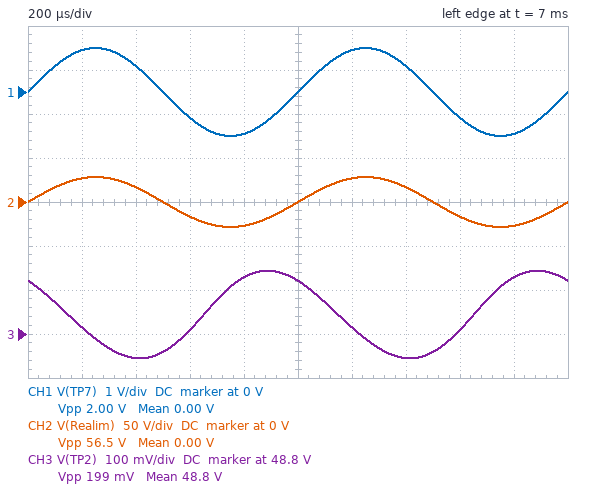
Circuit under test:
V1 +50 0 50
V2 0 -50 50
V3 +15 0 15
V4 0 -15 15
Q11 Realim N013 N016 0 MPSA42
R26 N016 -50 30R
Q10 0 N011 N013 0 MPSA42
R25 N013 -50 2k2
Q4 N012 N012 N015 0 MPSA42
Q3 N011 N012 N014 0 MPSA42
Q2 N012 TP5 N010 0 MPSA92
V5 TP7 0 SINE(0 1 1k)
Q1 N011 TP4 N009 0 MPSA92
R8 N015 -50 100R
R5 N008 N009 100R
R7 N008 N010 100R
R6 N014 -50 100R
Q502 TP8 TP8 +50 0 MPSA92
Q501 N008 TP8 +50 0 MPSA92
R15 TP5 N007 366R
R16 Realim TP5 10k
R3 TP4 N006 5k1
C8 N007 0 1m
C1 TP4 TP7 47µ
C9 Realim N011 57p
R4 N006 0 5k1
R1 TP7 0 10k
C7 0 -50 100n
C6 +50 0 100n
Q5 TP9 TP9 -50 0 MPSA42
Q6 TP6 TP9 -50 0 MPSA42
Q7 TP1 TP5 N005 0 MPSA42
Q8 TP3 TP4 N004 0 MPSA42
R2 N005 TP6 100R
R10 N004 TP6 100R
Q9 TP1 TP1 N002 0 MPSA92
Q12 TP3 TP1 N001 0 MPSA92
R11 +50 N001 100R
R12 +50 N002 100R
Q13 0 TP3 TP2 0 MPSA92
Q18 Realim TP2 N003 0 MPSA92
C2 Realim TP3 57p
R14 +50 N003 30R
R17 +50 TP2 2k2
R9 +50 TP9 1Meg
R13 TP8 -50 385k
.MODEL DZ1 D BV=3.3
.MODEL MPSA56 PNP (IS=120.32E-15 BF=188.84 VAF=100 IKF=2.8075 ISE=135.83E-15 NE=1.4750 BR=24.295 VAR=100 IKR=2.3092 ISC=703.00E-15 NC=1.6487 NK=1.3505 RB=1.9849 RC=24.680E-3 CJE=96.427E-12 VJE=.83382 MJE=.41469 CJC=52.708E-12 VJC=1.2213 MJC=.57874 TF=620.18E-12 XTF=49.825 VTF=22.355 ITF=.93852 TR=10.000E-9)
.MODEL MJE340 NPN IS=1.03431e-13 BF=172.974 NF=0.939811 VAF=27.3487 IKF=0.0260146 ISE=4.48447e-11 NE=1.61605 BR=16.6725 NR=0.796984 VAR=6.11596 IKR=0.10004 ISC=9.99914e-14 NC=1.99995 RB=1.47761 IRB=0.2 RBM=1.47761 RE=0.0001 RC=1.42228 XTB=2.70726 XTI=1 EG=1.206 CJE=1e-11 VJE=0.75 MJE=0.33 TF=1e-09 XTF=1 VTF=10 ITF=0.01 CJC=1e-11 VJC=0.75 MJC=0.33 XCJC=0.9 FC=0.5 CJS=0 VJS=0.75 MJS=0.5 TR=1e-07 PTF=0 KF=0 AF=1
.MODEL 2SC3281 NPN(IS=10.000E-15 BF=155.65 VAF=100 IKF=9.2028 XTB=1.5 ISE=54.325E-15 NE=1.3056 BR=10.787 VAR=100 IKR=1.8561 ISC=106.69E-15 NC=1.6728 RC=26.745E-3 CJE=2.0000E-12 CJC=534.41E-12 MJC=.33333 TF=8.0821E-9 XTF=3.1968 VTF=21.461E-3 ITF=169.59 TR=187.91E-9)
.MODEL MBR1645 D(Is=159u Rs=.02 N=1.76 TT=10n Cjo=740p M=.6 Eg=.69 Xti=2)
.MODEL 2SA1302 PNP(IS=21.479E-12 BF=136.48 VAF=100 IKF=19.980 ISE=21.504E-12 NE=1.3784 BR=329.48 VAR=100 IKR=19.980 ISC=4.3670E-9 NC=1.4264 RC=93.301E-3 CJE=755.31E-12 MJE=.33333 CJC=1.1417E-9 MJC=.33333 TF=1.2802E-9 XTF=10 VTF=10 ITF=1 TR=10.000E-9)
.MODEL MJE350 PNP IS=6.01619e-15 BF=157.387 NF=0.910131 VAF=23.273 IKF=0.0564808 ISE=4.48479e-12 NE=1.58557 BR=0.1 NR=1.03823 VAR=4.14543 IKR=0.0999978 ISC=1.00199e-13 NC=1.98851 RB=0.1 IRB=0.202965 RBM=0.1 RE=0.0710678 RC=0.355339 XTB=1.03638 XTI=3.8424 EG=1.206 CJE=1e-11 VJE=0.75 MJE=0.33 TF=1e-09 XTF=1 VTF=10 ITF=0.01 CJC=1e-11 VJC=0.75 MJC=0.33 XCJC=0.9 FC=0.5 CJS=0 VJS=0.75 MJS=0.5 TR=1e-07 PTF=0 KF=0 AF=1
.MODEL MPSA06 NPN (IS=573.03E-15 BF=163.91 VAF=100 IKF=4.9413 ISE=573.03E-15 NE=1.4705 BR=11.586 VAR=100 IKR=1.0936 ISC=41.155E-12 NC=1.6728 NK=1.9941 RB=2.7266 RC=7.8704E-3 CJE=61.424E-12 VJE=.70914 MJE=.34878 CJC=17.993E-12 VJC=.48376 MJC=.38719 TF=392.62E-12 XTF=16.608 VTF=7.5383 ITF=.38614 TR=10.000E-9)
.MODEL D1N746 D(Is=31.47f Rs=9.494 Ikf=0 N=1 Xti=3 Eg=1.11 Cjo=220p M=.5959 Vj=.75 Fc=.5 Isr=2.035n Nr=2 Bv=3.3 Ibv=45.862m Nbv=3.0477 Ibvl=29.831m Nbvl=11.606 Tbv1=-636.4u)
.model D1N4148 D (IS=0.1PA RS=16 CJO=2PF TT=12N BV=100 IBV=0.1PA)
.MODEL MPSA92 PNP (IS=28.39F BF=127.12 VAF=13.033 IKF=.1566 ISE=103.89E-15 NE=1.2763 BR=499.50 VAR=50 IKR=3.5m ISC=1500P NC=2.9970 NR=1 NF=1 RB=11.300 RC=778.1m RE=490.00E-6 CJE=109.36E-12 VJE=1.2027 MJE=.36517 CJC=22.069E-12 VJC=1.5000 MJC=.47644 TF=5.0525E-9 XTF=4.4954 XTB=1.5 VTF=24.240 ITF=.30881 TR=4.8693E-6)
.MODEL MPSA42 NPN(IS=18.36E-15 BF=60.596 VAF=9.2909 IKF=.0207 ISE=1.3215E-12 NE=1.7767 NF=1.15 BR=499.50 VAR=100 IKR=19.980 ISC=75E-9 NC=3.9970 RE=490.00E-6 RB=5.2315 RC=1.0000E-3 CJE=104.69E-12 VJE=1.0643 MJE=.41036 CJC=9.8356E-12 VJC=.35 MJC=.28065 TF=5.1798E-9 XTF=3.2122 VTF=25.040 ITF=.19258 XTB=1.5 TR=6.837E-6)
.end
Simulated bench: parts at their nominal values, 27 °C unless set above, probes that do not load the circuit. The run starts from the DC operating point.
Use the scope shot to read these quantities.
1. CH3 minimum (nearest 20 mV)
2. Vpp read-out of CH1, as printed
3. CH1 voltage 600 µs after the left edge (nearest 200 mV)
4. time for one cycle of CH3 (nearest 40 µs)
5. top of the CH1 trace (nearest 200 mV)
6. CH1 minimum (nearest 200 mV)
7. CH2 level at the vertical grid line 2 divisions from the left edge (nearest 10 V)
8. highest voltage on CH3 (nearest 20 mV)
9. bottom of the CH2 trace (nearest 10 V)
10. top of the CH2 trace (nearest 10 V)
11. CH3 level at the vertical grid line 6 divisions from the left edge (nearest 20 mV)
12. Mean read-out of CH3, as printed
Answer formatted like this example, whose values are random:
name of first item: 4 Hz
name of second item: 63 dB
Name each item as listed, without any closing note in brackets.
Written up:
CH3 minimum: 48.74 V
Vpp read-out of CH1, as printed: 2.00 V
CH1 voltage 600 µs after the left edge: -600 mV
time for one cycle of CH3: 1.00 ms
top of the CH1 trace: 1.0 V
CH1 minimum: -1.0 V
CH2 level at the vertical grid line 2 divisions from the left edge: 20 V
highest voltage on CH3: 48.94 V
bottom of the CH2 trace: -30 V
top of the CH2 trace: 30 V
CH3 level at the vertical grid line 6 divisions from the left edge: 48.82 V
Mean read-out of CH3, as printed: 48.8 V
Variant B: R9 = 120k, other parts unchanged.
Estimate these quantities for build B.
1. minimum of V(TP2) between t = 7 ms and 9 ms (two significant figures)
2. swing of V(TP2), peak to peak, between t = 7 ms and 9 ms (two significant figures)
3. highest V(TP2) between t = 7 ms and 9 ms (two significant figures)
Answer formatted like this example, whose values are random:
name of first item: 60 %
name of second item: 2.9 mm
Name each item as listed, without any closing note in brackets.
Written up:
minimum of V(TP2) between t = 7 ms and 9 ms: 47 V
swing of V(TP2), peak to peak, between t = 7 ms and 9 ms: 220 mV
highest V(TP2) between t = 7 ms and 9 ms: 48 V
